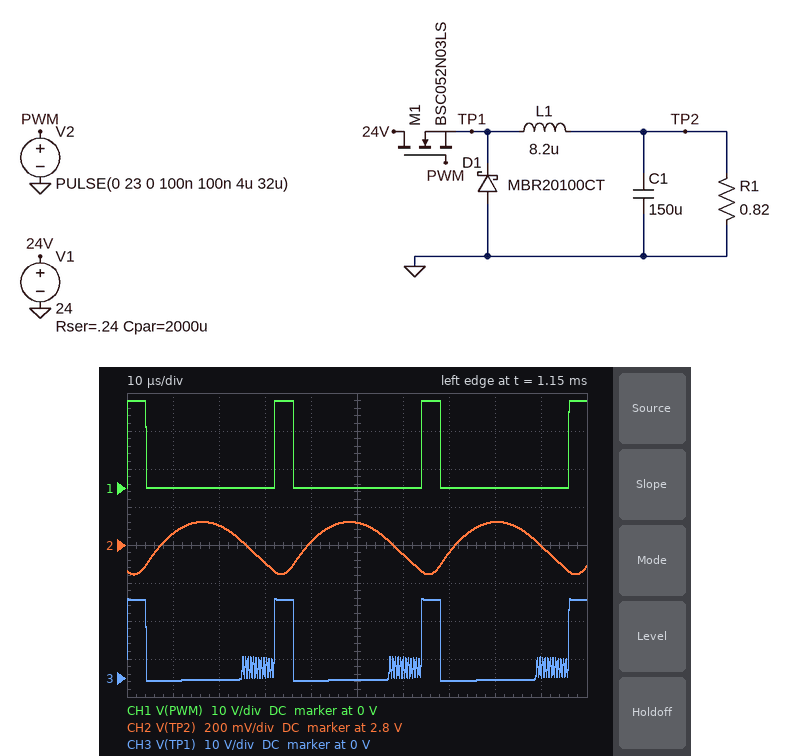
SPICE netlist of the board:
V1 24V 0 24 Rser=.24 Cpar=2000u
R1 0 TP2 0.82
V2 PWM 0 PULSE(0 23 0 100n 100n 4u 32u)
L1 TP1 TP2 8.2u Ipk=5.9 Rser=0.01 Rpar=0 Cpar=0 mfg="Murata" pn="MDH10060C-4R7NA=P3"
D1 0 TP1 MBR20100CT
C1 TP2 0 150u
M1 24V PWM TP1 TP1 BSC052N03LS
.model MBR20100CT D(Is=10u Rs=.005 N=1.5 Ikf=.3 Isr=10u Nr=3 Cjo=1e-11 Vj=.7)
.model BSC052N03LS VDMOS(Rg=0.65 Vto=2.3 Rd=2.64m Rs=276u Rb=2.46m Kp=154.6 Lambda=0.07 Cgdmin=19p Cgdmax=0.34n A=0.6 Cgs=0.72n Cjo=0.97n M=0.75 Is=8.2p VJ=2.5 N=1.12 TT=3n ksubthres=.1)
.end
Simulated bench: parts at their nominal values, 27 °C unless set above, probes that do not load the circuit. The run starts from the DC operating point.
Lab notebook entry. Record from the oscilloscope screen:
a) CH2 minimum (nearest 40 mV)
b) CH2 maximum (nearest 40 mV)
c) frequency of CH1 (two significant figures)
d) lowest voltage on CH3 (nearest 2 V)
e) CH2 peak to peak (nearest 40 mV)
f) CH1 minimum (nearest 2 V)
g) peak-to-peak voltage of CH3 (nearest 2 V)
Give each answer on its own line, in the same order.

2.64 V
2.92 V
31 kHz
0 V
280 mV
0 V
22 V
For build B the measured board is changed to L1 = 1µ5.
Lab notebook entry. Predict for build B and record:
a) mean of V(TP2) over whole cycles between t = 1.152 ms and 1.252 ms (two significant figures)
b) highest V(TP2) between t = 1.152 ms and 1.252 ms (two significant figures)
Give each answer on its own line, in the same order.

6.1 V
6.6 V
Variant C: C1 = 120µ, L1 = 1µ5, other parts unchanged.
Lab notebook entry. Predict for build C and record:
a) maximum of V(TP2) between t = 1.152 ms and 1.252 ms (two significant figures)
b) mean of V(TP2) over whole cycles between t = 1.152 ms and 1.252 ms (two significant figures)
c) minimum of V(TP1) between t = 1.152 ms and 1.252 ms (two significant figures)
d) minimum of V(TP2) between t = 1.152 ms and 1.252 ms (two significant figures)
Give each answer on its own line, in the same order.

6.7 V
6.1 V
-980 mV
5.4 V
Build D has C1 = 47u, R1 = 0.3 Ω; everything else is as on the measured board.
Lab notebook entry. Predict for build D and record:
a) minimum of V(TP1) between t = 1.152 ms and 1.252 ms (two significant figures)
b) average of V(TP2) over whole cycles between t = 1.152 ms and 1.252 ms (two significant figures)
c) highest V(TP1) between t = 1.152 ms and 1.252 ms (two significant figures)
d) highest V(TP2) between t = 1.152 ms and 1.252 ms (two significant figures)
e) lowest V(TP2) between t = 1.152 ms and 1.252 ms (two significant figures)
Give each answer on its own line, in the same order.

-740 mV
2.0 V
21 V
2.3 V
1.5 V
